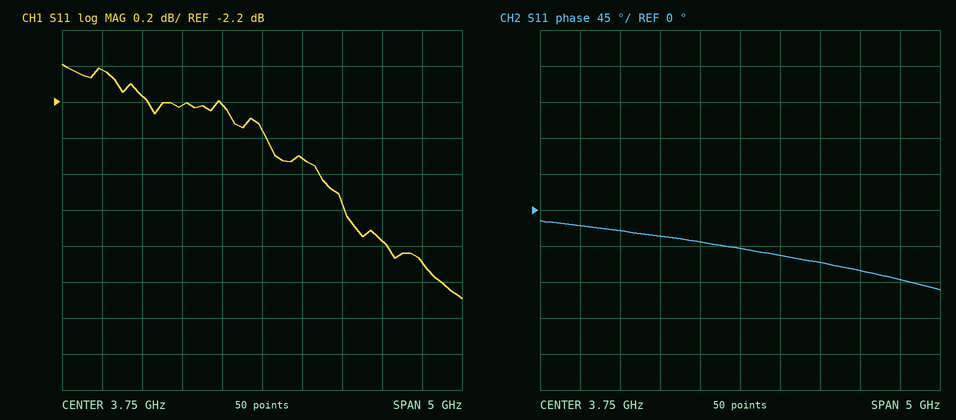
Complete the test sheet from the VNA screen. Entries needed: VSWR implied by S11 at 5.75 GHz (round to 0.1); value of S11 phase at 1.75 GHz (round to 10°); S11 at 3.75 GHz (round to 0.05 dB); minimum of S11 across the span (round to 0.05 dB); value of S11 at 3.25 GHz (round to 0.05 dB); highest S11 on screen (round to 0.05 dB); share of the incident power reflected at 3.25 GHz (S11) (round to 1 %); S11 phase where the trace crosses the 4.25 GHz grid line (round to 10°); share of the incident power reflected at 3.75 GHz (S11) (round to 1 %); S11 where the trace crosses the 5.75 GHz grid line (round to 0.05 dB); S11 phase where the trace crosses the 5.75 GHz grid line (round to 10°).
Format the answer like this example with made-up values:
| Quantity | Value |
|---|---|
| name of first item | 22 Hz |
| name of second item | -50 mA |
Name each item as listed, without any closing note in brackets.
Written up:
| Quantity | Value |
|---|---|
| VSWR implied by S11 at 5.75 GHz | 5.7 |
| value of S11 phase at 1.75 GHz | -20° |
| S11 at 3.75 GHz | -2.35 dB |
| minimum of S11 across the span | -3.30 dB |
| value of S11 at 3.25 GHz | -2.20 dB |
| highest S11 on screen | -2.00 dB |
| share of the incident power reflected at 3.25 GHz (S11) | 60 % |
| S11 phase where the trace crosses the 4.25 GHz grid line | -60° |
| share of the incident power reflected at 3.75 GHz (S11) | 58 % |
| S11 where the trace crosses the 5.75 GHz grid line | -3.10 dB |
| S11 phase where the trace crosses the 5.75 GHz grid line | -90° |
